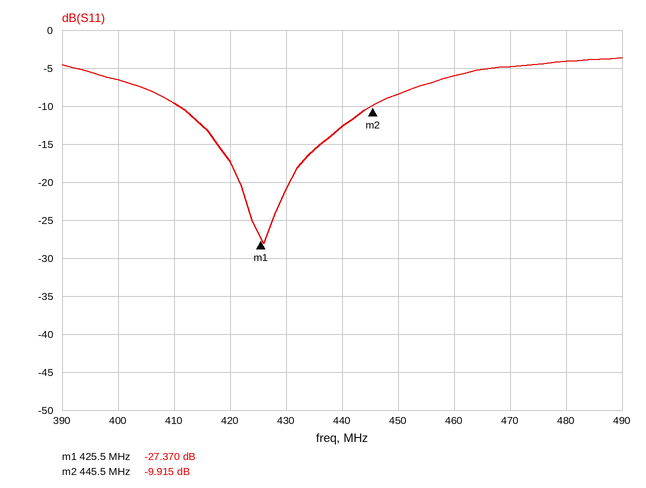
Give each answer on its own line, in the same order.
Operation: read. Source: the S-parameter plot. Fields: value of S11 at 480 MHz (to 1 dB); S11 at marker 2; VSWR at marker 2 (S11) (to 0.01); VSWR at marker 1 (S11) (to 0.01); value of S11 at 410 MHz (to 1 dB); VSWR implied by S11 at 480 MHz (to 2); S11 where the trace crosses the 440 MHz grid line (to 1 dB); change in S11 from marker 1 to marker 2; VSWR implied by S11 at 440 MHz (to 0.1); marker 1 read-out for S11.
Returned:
-4 dB
-9.915 dB
1.94
1.09
-10 dB
4
-13 dB
17.455 dB
1.6
-27.370 dB
